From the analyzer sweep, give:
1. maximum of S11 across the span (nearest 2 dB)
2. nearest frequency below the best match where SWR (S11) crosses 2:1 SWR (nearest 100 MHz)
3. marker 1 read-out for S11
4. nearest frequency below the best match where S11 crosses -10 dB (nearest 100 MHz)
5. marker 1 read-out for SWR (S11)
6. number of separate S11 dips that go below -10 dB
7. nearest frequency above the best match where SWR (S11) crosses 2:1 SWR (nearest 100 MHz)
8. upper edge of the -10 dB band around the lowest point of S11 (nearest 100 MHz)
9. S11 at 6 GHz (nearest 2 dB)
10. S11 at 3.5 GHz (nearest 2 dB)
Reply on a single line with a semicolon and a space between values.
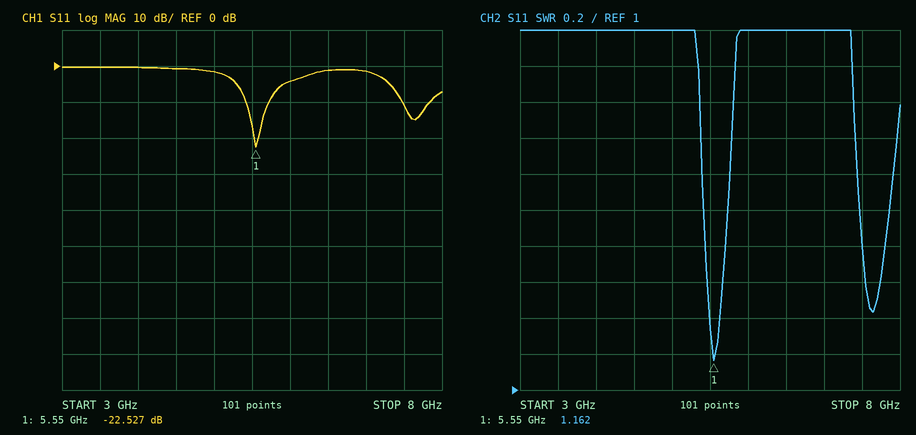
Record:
0 dB; 5.4 GHz; -22.527 dB; 5.4 GHz; 1.162; 2; 5.7 GHz; 5.7 GHz; -4 dB; 0 dB
